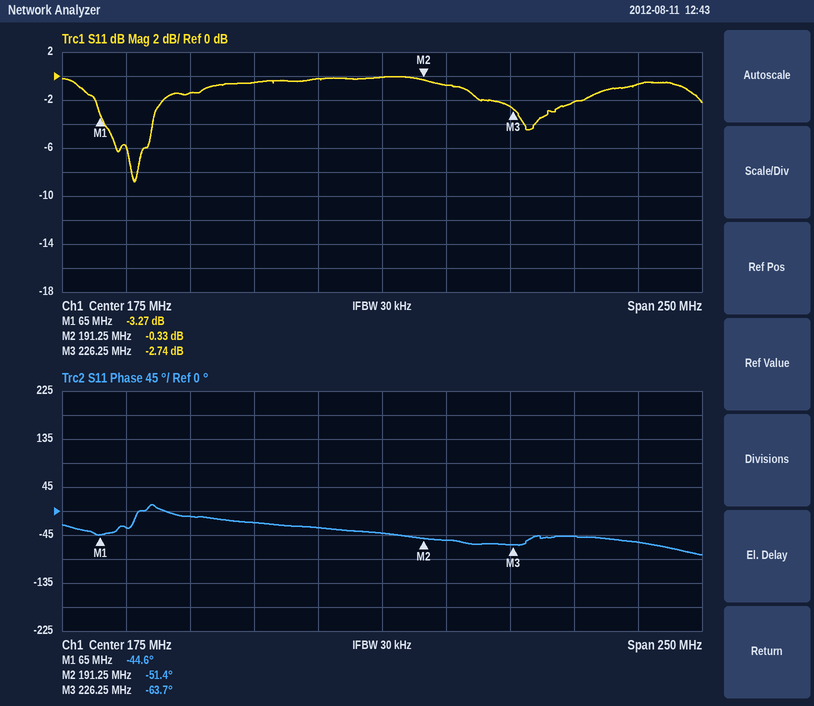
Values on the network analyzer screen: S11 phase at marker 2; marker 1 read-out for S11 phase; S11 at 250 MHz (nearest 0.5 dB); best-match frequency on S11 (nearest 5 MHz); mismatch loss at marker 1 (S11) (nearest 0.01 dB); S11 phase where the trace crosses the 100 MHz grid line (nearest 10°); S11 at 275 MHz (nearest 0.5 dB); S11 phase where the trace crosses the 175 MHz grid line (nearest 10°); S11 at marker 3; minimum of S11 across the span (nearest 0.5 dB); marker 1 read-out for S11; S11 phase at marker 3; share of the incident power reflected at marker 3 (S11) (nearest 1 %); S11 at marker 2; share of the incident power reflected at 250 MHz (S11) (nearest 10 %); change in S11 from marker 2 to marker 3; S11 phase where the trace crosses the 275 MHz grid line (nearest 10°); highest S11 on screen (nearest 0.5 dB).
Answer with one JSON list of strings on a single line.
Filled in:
["-51.4°", "-44.6°", "-2.0 dB", "80 MHz", "2.77 dB", "-10°", "-0.5 dB", "-40°", "-2.74 dB", "-9.0 dB", "-3.27 dB", "-63.7°", "53 %", "-0.33 dB", "60 %", "-2.41 dB", "-60°", "0.0 dB"]
